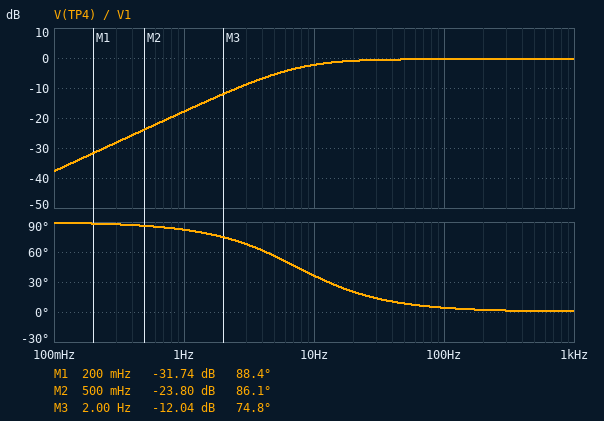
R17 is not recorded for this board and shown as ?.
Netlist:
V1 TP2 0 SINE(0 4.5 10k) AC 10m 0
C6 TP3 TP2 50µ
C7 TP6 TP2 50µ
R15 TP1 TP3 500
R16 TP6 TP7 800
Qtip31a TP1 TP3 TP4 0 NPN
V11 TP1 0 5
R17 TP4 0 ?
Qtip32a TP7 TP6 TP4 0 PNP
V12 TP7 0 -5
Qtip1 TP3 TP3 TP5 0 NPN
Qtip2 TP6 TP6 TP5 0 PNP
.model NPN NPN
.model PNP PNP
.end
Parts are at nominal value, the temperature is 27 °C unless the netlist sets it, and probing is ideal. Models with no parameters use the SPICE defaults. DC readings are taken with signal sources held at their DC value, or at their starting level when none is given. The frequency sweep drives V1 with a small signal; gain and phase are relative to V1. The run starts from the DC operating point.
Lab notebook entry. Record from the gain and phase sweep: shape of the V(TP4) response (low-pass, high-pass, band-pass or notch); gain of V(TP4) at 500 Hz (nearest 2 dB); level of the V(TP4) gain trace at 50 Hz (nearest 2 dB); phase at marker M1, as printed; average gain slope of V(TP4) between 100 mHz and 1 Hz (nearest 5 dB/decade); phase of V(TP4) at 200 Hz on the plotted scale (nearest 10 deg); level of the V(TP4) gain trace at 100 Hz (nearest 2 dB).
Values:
high-pass
0 dB
0 dB
88.4 deg
20 dB/decade
0 deg
0 dB
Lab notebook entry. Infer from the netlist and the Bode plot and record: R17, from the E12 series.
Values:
6.8 Ω
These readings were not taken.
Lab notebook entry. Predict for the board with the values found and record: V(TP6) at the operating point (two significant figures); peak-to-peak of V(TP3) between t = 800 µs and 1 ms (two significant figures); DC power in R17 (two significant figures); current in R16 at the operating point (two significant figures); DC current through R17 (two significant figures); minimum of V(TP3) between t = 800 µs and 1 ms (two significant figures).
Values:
-130 mV
9.0 V
56 mW
6.1 mA
91 mA
-3.1 V
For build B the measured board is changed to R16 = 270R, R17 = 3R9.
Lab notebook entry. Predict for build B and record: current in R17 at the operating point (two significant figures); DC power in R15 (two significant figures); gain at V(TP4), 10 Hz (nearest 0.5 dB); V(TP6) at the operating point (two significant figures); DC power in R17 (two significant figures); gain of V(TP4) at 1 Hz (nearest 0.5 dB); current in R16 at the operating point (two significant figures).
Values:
210 mA
51 mW
-4.5 dB
-1.7 V
170 mW
-22.5 dB
12 mA
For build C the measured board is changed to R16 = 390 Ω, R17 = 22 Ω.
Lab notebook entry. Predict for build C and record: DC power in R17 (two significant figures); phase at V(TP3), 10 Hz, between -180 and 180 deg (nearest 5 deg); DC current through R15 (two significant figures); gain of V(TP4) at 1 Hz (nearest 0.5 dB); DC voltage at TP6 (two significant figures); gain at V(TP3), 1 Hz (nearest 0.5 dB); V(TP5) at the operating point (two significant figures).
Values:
9.1 mW
40 deg
9.3 mA
-18.5 dB
-1.3 V
-18.0 dB
-470 mV
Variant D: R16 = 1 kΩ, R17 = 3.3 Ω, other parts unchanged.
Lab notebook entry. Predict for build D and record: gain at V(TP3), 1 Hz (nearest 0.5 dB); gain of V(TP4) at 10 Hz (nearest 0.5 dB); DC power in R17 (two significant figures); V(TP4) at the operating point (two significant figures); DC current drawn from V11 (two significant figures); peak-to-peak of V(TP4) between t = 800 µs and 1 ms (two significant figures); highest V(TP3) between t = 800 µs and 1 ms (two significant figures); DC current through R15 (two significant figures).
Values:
-19.5 dB
-3.0 dB
130 mW
650 mV
200 mA
8.6 V
5.9 V
6.9 mA
